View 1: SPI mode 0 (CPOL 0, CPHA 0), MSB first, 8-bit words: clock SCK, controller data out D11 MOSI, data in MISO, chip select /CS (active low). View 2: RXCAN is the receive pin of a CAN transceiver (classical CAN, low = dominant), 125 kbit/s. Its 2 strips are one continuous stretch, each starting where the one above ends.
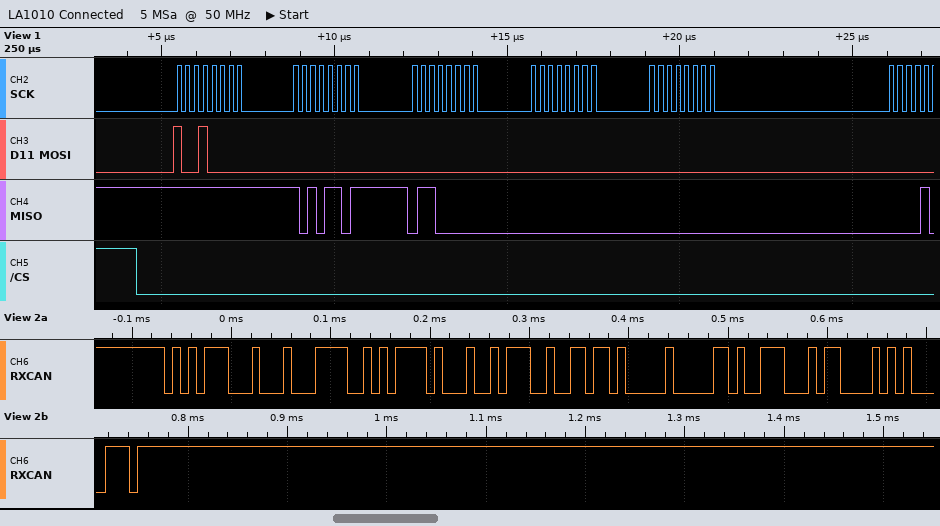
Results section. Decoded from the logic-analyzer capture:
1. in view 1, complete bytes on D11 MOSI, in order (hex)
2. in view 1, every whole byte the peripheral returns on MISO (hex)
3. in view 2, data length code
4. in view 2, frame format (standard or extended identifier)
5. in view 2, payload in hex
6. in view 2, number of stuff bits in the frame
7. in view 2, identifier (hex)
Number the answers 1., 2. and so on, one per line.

1. 0x90 0x00 0x00 0x00 0x00
2. 0xFF 0xAD 0x60 0x00 0x00
3. 8
4. standard
5. F2 BD 12 E4 DA 00 53 8B
6. 2
7. 0x571
